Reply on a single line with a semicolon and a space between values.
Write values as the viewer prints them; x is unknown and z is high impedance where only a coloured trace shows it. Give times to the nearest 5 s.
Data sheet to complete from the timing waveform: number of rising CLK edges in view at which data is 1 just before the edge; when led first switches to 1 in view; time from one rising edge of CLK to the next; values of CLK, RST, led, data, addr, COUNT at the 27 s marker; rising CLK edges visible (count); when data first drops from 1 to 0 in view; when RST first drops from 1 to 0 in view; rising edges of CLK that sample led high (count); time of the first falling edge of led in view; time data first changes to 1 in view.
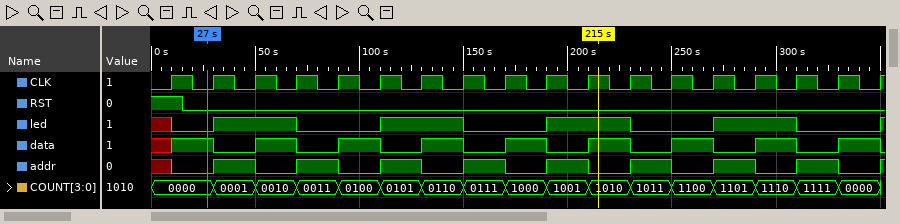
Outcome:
9; 30 s; 20 s; CLK=0, RST=0, led=0, data=1, addr=0, COUNT=0000; 18; 30 s; 15 s; 8; 70 s; 10 s
